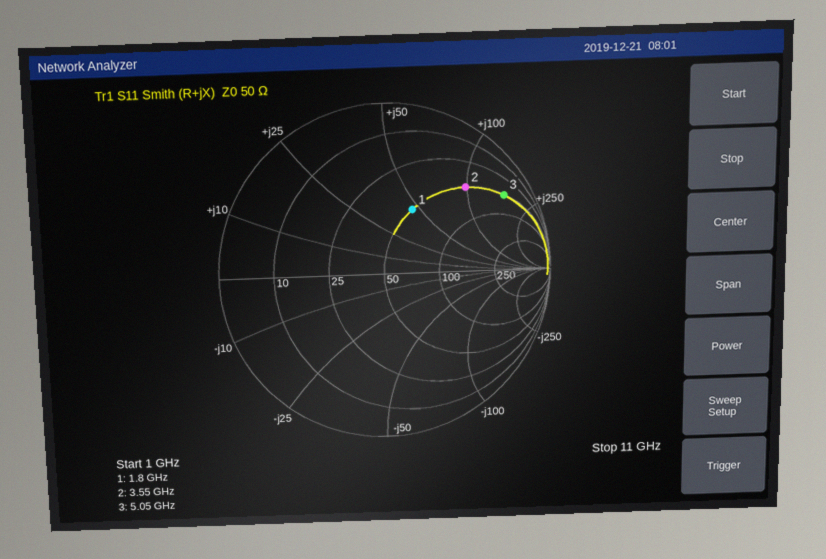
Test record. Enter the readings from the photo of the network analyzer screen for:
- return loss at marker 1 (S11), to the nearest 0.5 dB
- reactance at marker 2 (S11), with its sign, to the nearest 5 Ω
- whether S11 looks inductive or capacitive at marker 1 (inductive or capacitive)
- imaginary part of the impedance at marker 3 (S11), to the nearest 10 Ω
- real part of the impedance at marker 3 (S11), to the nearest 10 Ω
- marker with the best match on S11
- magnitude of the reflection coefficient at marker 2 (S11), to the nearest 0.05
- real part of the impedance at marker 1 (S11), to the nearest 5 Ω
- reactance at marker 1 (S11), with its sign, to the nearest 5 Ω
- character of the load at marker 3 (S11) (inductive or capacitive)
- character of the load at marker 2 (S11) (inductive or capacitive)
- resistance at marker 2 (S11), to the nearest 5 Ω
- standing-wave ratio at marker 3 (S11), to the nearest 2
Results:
7.5 dB
+100 Ω
inductive
+160 Ω
50 Ω
marker 1
0.70
50 Ω
+45 Ω
inductive
inductive
50 Ω
12
